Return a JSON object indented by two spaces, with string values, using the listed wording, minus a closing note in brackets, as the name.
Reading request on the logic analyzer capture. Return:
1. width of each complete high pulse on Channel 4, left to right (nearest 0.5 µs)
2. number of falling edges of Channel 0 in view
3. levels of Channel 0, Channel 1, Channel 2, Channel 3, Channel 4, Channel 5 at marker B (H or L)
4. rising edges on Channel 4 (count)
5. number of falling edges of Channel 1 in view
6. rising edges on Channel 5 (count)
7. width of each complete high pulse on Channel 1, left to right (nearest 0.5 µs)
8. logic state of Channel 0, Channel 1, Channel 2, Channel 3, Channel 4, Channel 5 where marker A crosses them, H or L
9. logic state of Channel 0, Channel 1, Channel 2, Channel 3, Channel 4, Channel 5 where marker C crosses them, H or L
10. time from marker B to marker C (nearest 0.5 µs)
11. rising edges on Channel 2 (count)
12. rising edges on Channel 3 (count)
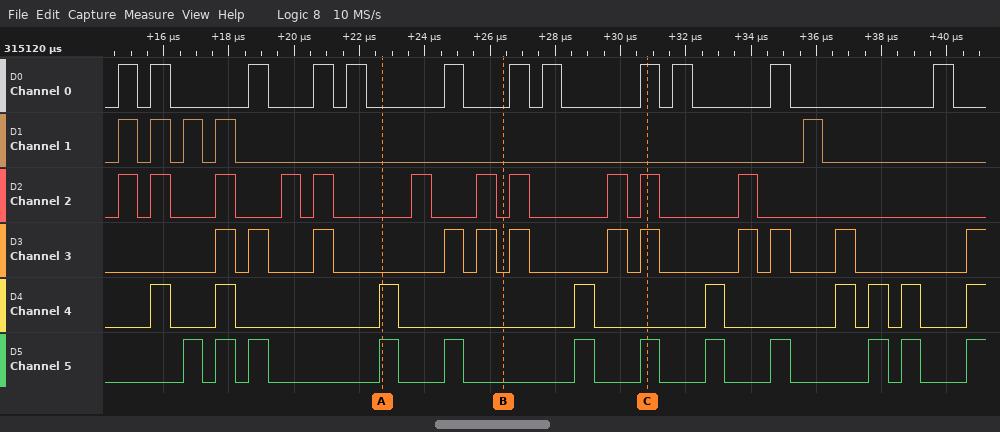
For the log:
{
  "width of each complete high pulse on Channel 4, left to right": "0.5 µs, 0.5 µs, 0.5 µs, 0.5 µs, 0.5 µs, 0.5 µs, 0.5 µs, 0.5 µs",
  "number of falling edges of Channel 0 in view": "12",
  "levels of Channel 0, Channel 1, Channel 2, Channel 3, Channel 4, Channel 5 at marker B": "Channel 0=L, Channel 1=L, Channel 2=L, Channel 3=L, Channel 4=L, Channel 5=L",
  "rising edges on Channel 4": "9",
  "number of falling edges of Channel 1 in view": "5",
  "rising edges on Channel 5": "12",
  "width of each complete high pulse on Channel 1, left to right": "0.5 µs, 0.5 µs, 0.5 µs, 0.5 µs, 0.5 µs",
  "logic state of Channel 0, Channel 1, Channel 2, Channel 3, Channel 4, Channel 5 where marker A crosses them, H or L": "Channel 0=L, Channel 1=L, Channel 2=L, Channel 3=L, Channel 4=H, Channel 5=H",
  "logic state of Channel 0, Channel 1, Channel 2, Channel 3, Channel 4, Channel 5 where marker C crosses them, H or L": "Channel 0=H, Channel 1=L, Channel 2=H, Channel 3=H, Channel 4=L, Channel 5=H",
  "time from marker B to marker C": "4.5 µs",
  "rising edges on Channel 2": "11",
  "rising edges on Channel 3": "12"
}
